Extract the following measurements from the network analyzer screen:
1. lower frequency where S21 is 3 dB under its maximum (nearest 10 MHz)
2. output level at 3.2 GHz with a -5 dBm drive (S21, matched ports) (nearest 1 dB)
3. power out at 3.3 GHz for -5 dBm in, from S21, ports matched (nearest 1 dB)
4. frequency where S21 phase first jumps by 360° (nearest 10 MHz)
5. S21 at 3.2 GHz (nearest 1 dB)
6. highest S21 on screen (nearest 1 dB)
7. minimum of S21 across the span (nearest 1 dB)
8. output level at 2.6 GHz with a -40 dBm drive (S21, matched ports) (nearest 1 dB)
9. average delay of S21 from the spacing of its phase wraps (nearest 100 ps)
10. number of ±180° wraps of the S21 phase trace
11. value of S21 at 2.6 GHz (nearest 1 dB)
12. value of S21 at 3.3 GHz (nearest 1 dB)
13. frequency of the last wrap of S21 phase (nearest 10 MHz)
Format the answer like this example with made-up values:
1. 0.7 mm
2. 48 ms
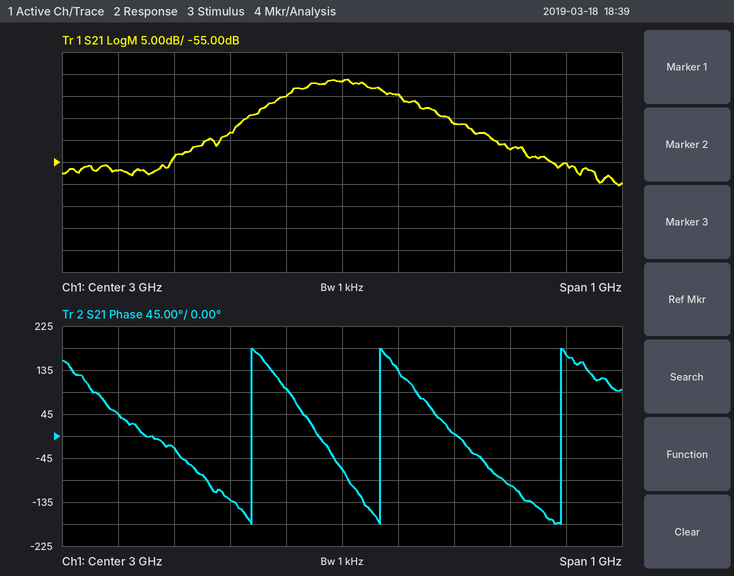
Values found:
1. 2.91 GHz
2. -51 dBm
3. -57 dBm
4. 2.84 GHz
5. -46 dB
6. -36 dB
7. -60 dB
8. -97 dBm
9. 3.6 ns
10. 3
11. -57 dB
12. -52 dB
13. 3.39 GHz
